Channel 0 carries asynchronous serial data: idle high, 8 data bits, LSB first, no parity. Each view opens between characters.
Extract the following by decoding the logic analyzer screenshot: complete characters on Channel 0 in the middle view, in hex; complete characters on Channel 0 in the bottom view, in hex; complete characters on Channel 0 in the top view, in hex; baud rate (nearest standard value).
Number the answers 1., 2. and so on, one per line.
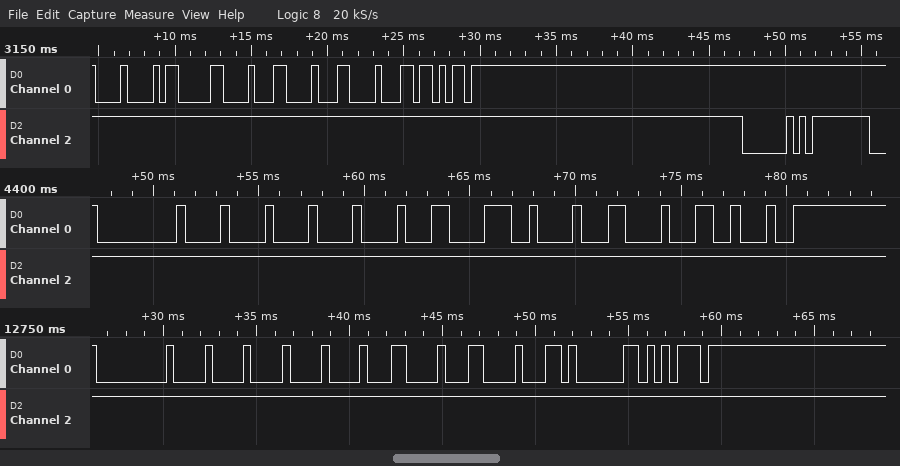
1. 00, 08, 08, 88, 38, 88, 88, 22
2. 00, 08, 08, 88, 88, 88, 81, 75
3. 08, 83, 88, 88, 88, 6B
4. 2400 baud
